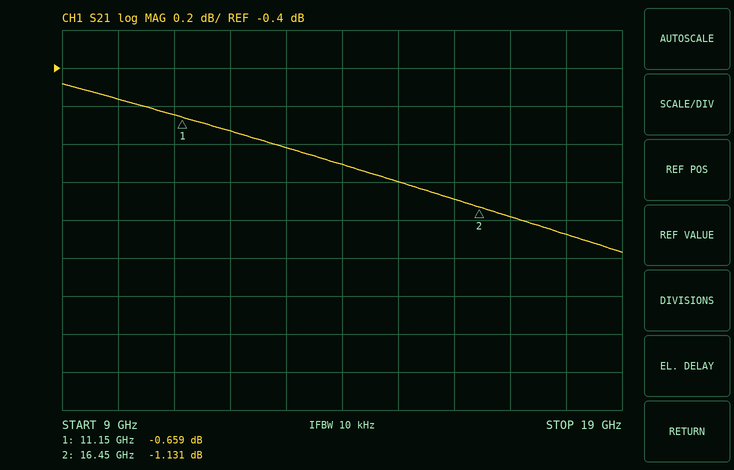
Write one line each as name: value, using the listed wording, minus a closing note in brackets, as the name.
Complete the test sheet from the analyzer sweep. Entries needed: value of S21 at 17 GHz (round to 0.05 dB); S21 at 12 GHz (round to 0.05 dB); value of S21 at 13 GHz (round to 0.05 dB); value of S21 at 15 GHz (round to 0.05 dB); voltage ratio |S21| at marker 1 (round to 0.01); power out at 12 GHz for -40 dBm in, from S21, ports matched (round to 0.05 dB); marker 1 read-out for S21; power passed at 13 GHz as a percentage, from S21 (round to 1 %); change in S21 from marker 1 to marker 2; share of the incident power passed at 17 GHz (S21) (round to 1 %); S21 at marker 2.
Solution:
value of S21 at 17 GHz: -1.20 dB
S21 at 12 GHz: -0.75 dB
value of S21 at 13 GHz: -0.80 dB
value of S21 at 15 GHz: -1.00 dB
voltage ratio |S21| at marker 1: 0.93
power out at 12 GHz for -40 dBm in, from S21, ports matched: -40.75 dBm
marker 1 read-out for S21: -0.659 dB
power passed at 13 GHz as a percentage, from S21: 83 %
change in S21 from marker 1 to marker 2: -0.472 dB
share of the incident power passed at 17 GHz (S21): 76 %
S21 at marker 2: -1.131 dB
